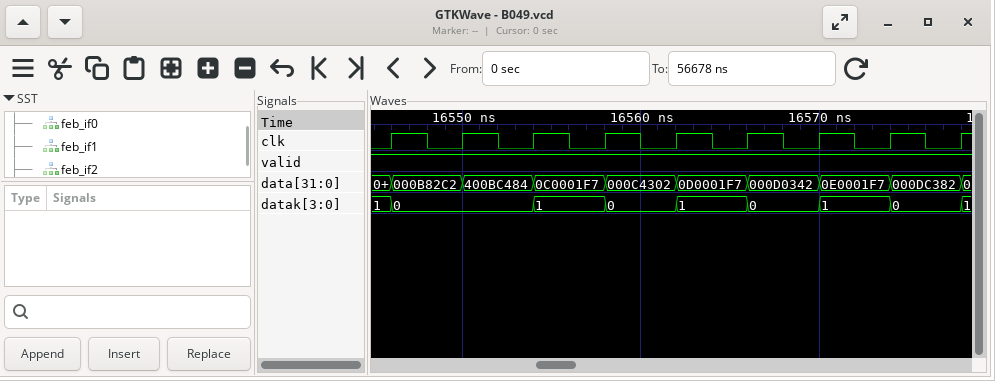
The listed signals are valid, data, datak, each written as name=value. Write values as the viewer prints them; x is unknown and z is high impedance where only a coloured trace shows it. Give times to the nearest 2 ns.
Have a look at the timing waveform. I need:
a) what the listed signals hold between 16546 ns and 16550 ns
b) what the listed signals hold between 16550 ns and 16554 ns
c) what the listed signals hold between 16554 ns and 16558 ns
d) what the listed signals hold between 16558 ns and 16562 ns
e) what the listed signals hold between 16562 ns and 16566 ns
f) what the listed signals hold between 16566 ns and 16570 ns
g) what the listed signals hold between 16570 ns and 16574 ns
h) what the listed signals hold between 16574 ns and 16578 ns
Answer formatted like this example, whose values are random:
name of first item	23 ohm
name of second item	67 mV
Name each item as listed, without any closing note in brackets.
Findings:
what the listed signals hold between 16546 ns and 16550 ns	valid=1, data=000B82C2, datak=0
what the listed signals hold between 16550 ns and 16554 ns	valid=1, data=400BC484, datak=0
what the listed signals hold between 16554 ns and 16558 ns	valid=1, data=0C0001F7, datak=1
what the listed signals hold between 16558 ns and 16562 ns	valid=1, data=000C4302, datak=0
what the listed signals hold between 16562 ns and 16566 ns	valid=1, data=0D0001F7, datak=1
what the listed signals hold between 16566 ns and 16570 ns	valid=1, data=000D0342, datak=0
what the listed signals hold between 16570 ns and 16574 ns	valid=1, data=0E0001F7, datak=1
what the listed signals hold between 16574 ns and 16578 ns	valid=1, data=000DC382, datak=0
